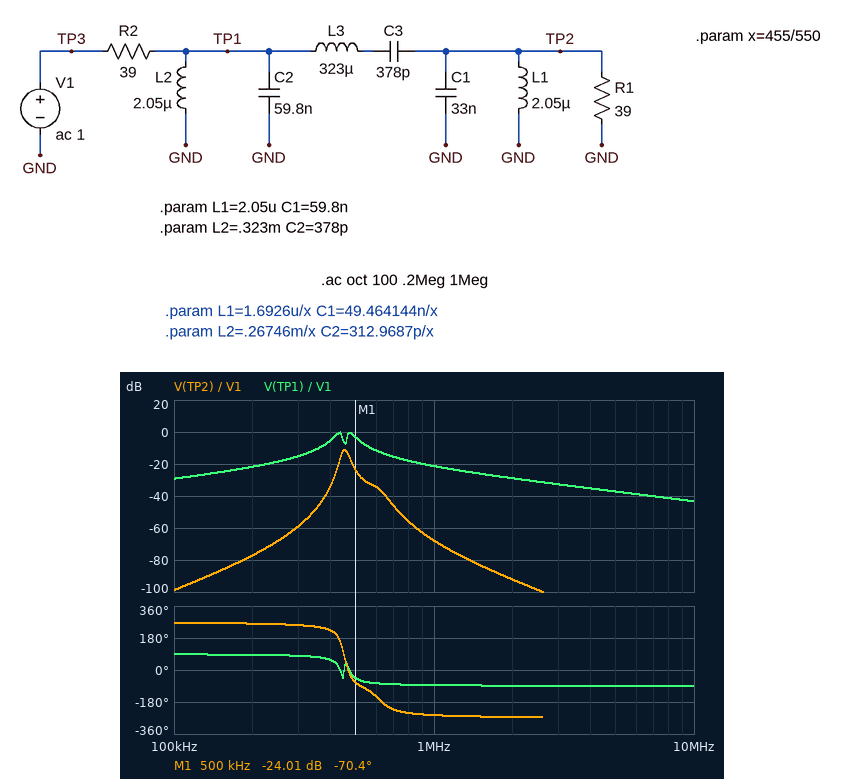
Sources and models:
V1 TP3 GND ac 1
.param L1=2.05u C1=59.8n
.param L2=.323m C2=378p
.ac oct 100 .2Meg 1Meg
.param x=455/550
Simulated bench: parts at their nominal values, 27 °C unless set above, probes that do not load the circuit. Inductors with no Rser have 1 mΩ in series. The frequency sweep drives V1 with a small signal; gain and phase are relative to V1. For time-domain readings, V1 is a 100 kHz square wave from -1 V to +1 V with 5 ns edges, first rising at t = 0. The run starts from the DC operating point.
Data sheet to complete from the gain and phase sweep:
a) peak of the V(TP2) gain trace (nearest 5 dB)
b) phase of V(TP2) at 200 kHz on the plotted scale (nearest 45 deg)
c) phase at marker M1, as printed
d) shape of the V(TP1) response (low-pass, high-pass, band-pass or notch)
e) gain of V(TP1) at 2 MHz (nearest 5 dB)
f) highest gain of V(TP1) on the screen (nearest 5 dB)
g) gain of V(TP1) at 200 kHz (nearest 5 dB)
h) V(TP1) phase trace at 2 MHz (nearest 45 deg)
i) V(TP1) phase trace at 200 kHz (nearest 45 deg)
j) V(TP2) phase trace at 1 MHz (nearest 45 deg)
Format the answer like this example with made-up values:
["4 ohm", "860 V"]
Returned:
["-10 dB", "270 deg", "-70.4 deg", "band-pass", "-30 dB", "0 dB", "-20 dB", "-90 deg", "90 deg", "-270 deg"]
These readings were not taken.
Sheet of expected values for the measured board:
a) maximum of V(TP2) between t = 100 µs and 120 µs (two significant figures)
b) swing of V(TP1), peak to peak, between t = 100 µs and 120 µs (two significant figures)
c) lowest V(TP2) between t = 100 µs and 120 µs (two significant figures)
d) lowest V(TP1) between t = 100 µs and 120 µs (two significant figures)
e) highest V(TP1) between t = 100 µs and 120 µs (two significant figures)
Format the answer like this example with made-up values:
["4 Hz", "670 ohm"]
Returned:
["16 mV", "550 mV", "-16 mV", "-280 mV", "280 mV"]
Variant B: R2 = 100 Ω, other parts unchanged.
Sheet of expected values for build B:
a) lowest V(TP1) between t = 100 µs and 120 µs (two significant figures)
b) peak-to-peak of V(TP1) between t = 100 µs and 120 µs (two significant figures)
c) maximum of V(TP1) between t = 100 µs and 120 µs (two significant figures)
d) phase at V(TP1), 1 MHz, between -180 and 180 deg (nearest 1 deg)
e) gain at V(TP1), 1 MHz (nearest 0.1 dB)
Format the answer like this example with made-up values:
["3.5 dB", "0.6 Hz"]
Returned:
["-110 mV", "220 mV", "110 mV", "-88 deg", "-29.5 dB"]
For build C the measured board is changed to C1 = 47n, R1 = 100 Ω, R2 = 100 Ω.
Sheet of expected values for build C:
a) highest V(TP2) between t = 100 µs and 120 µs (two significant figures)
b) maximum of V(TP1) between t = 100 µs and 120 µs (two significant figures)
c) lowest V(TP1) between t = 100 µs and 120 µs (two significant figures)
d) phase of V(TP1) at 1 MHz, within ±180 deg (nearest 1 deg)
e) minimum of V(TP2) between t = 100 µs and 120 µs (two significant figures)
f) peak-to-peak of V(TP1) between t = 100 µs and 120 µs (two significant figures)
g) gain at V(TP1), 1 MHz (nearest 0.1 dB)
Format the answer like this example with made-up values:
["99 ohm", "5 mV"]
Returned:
["29 mV", "110 mV", "-110 mV", "-88 deg", "-29 mV", "220 mV", "-29.5 dB"]
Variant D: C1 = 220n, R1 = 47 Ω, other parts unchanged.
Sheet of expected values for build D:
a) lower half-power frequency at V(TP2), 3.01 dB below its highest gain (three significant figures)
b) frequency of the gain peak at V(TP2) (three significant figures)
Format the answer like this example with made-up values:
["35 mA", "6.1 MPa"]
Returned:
["443 kHz", "456 kHz"]
